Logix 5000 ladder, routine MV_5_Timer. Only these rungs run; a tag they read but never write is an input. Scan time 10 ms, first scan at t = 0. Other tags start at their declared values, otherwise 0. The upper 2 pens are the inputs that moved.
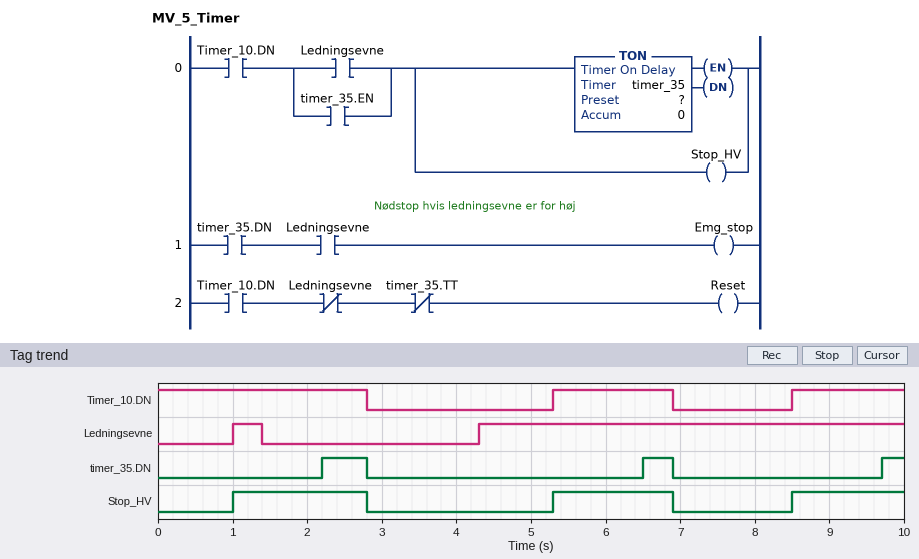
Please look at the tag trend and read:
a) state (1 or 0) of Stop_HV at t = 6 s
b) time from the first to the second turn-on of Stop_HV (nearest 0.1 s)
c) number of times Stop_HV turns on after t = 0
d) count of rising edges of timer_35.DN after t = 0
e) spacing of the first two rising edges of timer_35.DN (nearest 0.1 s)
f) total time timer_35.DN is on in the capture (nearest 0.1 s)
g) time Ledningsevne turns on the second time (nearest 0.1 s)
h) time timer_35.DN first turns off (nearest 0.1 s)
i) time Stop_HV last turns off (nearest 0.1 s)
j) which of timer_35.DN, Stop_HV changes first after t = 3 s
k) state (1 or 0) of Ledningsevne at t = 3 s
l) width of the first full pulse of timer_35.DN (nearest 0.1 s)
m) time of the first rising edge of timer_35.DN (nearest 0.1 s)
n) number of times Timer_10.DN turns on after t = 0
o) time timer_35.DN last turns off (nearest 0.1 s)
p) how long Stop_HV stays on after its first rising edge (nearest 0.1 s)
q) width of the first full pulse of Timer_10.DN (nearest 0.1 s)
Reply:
1
4.3 s
3
3
4.3 s
1.3 s
4.3 s
2.8 s
6.9 s
Stop_HV
0
0.6 s
2.2 s
2
6.9 s
1.8 s
1.6 s
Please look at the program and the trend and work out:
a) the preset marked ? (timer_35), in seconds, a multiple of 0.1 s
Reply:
1.2 s
